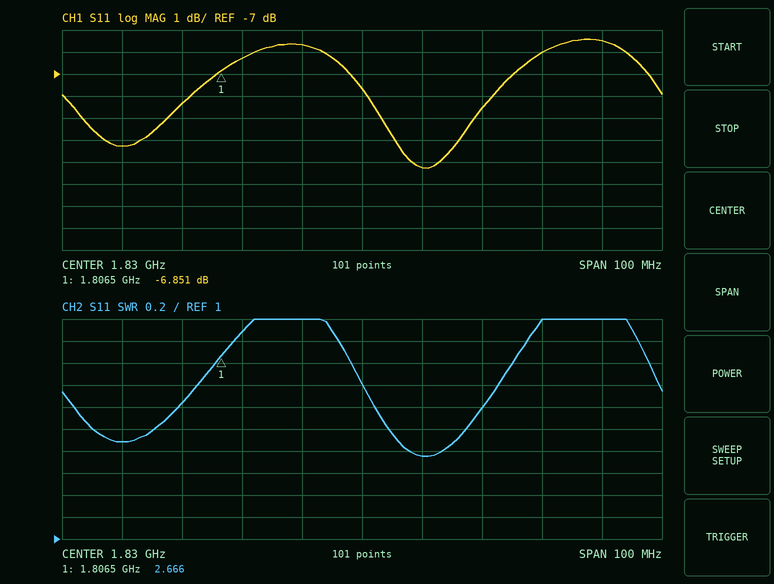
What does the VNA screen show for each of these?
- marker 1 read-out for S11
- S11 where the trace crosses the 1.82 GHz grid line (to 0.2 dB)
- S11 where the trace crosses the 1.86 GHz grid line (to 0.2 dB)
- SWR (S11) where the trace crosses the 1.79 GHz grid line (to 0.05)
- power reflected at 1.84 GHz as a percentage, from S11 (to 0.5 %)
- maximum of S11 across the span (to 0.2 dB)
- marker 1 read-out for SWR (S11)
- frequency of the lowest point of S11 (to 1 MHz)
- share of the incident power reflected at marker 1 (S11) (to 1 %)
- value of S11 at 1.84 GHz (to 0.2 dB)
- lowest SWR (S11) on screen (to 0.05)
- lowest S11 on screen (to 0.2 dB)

-6.851 dB
-5.6 dB
-6.0 dB
1.90
7.5 %
-5.4 dB
2.666
1.841 GHz
21 %
-11.2 dB
1.75
-11.2 dB
